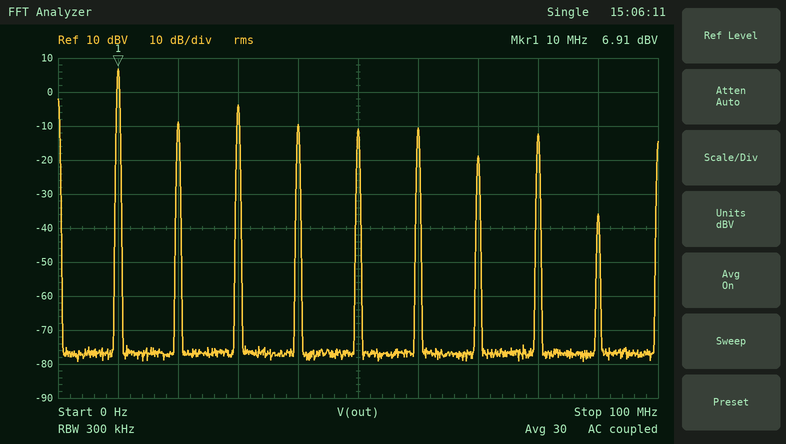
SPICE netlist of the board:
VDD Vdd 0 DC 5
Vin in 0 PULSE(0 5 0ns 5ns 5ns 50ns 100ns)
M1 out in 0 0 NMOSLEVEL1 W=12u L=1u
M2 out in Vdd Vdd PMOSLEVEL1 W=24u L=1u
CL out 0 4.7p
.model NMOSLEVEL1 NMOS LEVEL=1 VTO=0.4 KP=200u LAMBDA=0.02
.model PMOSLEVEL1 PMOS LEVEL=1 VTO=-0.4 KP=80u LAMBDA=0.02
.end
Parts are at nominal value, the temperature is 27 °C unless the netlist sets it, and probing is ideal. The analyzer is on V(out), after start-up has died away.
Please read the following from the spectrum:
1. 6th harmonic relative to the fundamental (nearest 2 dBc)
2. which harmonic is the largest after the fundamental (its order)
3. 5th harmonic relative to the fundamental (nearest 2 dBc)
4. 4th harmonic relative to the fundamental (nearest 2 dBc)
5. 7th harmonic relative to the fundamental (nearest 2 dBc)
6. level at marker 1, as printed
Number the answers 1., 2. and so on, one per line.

1. -18 dBc
2. 3
3. -18 dBc
4. -16 dBc
5. -26 dBc
6. 6.91 dBV
